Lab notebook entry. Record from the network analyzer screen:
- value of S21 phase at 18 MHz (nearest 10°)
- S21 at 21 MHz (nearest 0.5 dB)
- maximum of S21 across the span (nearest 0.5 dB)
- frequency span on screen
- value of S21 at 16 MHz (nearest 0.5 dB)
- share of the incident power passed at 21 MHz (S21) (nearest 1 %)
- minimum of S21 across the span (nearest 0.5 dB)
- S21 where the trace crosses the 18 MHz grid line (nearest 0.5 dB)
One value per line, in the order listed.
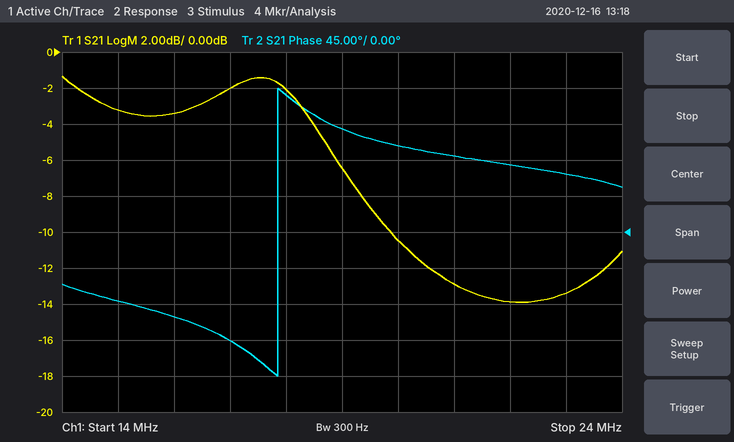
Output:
170°
-13.0 dB
-1.5 dB
10 MHz
-3.5 dB
5 %
-14.0 dB
-2.0 dB
